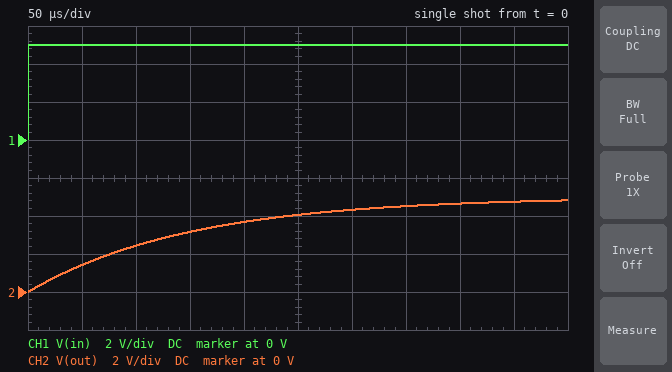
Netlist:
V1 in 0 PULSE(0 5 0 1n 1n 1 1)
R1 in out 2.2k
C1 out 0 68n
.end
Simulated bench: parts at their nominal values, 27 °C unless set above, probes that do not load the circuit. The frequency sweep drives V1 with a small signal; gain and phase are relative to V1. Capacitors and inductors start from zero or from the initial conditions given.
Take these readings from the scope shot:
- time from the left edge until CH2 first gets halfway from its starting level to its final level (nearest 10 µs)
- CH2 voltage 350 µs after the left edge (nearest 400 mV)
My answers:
100 µs
4.4 V
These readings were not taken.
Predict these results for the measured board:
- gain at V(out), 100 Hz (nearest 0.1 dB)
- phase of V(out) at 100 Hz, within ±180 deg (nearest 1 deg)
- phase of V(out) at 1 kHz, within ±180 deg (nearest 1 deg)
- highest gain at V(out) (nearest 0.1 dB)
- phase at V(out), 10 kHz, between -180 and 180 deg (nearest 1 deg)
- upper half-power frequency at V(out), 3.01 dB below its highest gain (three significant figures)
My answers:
0 dB
-5 deg
-43 deg
0 dB
-84 deg
1.06 kHz
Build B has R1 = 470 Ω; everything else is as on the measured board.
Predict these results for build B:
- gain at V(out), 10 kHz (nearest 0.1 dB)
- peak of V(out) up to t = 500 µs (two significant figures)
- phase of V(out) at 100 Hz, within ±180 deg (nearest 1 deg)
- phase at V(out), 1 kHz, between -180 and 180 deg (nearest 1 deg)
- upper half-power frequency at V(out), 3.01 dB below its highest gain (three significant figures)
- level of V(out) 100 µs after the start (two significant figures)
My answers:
-7.0 dB
5.0 V
-1 deg
-11 deg
4.98 kHz
4.8 V
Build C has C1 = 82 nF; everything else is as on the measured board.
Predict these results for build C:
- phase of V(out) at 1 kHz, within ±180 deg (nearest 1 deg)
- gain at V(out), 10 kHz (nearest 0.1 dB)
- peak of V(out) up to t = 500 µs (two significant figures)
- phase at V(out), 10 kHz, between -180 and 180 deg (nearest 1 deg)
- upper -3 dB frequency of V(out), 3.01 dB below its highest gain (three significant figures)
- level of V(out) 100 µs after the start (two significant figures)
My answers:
-49 deg
-21.1 dB
4.7 V
-85 deg
882 Hz
2.1 V
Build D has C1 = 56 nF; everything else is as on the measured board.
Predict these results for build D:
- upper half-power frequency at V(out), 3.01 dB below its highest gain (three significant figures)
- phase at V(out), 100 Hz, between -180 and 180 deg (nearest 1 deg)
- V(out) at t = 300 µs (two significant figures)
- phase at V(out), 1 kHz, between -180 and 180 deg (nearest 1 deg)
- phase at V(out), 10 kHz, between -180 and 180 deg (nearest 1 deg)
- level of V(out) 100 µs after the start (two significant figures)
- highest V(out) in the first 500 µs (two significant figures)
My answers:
1.29 kHz
-4 deg
4.6 V
-38 deg
-83 deg
2.8 V
4.9 V
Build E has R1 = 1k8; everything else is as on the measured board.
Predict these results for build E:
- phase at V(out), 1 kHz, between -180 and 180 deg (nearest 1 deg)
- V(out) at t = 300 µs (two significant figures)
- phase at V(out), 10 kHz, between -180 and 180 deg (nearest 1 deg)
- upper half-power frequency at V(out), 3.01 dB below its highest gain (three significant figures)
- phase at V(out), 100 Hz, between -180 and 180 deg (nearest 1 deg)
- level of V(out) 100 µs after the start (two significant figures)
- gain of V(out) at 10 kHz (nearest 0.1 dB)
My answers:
-38 deg
4.6 V
-83 deg
1.30 kHz
-4 deg
2.8 V
-17.8 dB
